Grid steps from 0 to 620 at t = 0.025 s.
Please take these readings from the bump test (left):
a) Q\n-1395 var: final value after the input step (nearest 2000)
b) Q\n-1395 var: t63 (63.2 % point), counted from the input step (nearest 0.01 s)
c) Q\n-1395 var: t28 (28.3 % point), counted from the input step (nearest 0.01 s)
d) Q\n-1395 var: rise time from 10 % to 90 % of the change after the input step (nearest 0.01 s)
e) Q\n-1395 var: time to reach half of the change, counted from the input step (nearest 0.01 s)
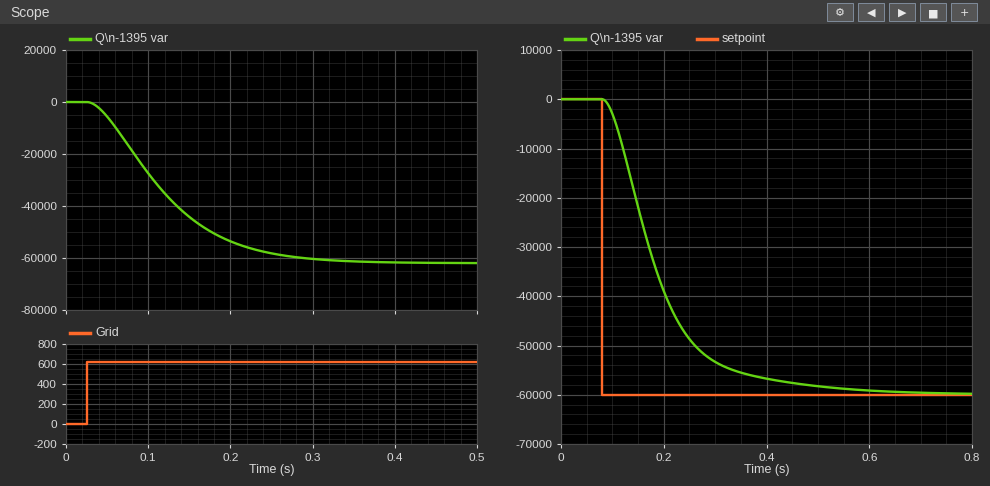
-62000
0.11 s
0.05 s
0.17 s
0.08 s
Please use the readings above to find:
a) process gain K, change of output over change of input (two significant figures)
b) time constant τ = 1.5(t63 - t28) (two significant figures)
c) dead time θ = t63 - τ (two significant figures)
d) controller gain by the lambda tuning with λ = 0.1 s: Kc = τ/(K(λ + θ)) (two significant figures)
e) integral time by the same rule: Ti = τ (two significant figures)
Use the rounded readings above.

-100
0.090 s
0.020 s
-0.0075
0.090 s
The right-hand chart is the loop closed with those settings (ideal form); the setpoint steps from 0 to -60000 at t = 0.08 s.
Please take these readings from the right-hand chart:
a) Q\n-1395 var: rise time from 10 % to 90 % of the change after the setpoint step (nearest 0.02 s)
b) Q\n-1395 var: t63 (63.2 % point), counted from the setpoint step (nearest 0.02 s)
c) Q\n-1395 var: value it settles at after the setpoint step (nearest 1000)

0.20 s
0.12 s
-60000
